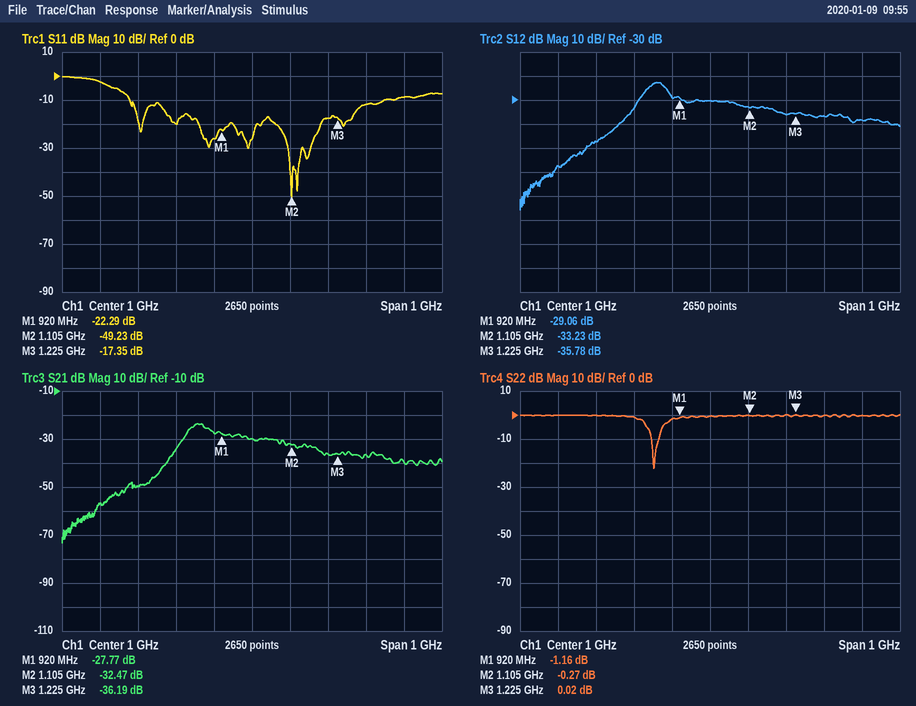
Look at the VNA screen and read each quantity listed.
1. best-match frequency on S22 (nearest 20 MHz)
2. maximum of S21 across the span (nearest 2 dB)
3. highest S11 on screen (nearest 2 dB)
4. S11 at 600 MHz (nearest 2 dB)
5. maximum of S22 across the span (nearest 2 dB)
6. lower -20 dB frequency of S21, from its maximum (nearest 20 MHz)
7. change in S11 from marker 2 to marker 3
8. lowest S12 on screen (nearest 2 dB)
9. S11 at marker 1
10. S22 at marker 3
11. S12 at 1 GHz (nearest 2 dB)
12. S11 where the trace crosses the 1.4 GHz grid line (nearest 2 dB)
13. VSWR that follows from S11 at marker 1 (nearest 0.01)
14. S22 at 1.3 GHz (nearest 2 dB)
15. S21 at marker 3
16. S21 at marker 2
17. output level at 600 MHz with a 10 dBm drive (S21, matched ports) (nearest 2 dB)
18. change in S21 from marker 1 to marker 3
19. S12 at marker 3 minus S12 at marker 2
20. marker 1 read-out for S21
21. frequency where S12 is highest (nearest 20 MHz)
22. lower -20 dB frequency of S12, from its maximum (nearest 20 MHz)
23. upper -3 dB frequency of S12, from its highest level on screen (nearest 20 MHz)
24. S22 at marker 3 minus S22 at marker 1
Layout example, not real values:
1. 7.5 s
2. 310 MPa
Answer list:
1. 860 MHz
2. -24 dB
3. 0 dB
4. -2 dB
5. 0 dB
6. 760 MHz
7. 31.88 dB
8. -76 dB
9. -22.29 dB
10. 0.02 dB
11. -30 dB
12. -8 dB
13. 1.17
14. 0 dB
15. -36.19 dB
16. -32.47 dB
17. -46 dBm
18. -8.42 dB
19. -2.55 dB
20. -27.77 dB
21. 860 MHz
22. 740 MHz
23. 880 MHz
24. 1.18 dB
